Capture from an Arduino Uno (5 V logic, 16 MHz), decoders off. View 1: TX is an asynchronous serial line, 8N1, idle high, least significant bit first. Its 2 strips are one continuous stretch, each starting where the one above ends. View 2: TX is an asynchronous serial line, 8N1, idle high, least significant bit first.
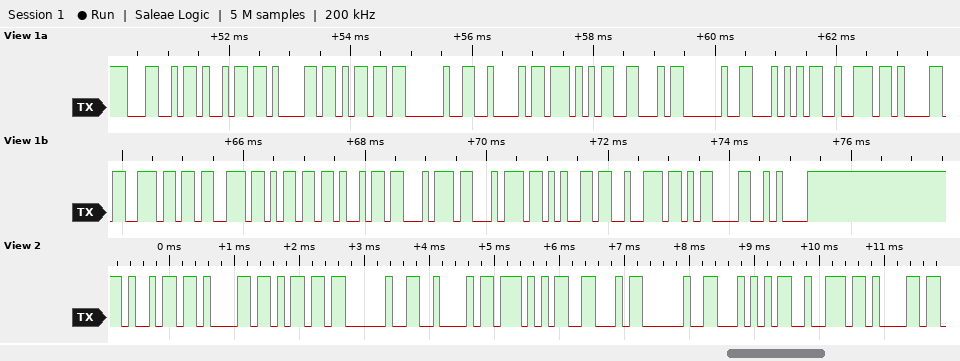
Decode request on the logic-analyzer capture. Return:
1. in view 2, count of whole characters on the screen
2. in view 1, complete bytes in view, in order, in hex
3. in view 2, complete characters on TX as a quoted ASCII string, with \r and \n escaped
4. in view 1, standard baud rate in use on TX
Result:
11
0x4C 0x69 0x61 0x6D 0x20 0x42 0x57 0x46 0x20 0x54 0x72 0x61 0x6E 0x73 0x6D 0x69 0x74 0x74 0x65 0x72 0x0D 0x0A
"iam BWF Tra"
9600 baud
